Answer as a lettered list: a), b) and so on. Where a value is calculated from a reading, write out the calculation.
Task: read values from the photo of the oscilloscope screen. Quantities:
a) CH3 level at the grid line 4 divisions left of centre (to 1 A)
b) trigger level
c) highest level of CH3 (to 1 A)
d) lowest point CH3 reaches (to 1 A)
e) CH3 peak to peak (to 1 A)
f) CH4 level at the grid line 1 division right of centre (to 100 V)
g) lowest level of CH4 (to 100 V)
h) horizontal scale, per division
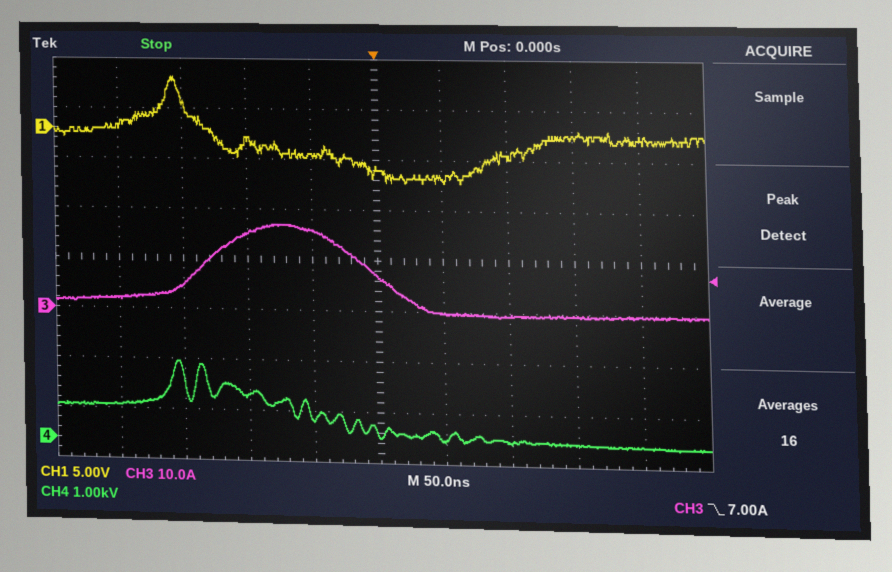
a) 2 A
b) 7.00 A
c) 17 A
d) -1 A
e) 17 A − (-1 A) = 18 A
f) 100 V
g) 0.0 kV
h) 50 ns
